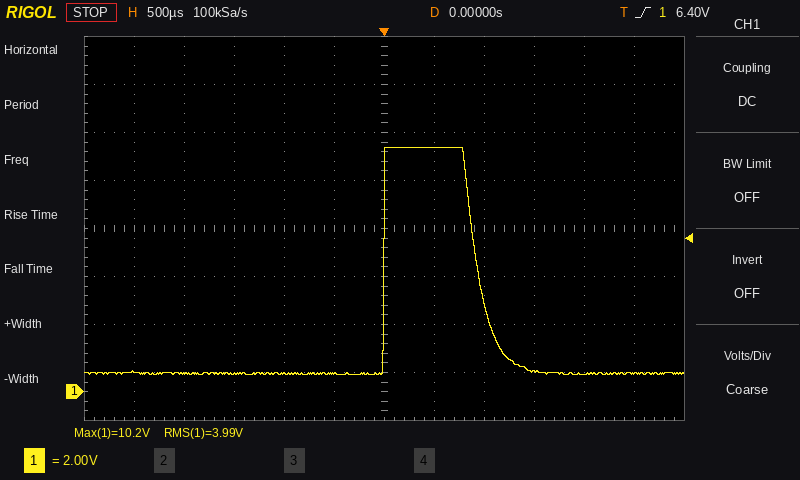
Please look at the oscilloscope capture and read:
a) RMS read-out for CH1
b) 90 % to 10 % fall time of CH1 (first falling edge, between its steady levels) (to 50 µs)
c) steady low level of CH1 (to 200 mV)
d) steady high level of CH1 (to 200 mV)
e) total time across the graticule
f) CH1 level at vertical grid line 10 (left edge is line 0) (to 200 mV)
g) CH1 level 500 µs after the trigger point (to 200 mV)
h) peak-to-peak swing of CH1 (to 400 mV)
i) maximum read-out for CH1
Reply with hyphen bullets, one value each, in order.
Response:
- 3.99 V
- 350 µs
- 800 mV
- 10.2 V
- 6 ms
- 800 mV
- 10.2 V
- 9.6 V
- 10.2 V
